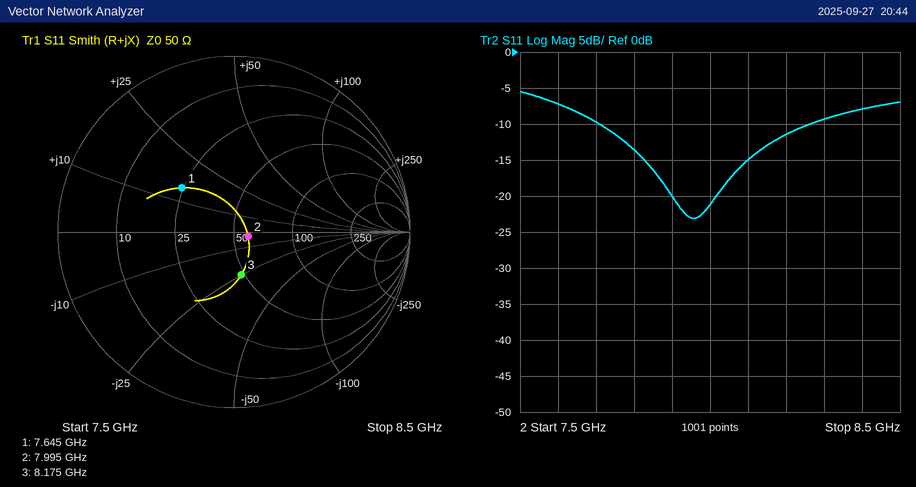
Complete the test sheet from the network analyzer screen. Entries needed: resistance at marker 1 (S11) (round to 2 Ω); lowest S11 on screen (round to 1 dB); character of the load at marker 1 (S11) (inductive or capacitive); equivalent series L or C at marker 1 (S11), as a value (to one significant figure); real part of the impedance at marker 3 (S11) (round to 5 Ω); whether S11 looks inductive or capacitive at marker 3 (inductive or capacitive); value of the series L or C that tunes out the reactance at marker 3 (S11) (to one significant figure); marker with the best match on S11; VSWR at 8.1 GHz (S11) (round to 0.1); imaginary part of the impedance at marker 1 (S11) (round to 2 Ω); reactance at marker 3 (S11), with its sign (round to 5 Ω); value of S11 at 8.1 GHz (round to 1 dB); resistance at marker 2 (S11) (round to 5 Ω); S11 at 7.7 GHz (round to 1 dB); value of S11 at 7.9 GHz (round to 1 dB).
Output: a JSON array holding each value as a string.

["24 Ω", "-23 dB", "inductive", "300 pH", "50 Ω", "capacitive", "500 pH", "marker 2", "1.4", "+14 Ω", "-25 Ω", "-15 dB", "60 Ω", "-10 dB", "-20 dB"]
